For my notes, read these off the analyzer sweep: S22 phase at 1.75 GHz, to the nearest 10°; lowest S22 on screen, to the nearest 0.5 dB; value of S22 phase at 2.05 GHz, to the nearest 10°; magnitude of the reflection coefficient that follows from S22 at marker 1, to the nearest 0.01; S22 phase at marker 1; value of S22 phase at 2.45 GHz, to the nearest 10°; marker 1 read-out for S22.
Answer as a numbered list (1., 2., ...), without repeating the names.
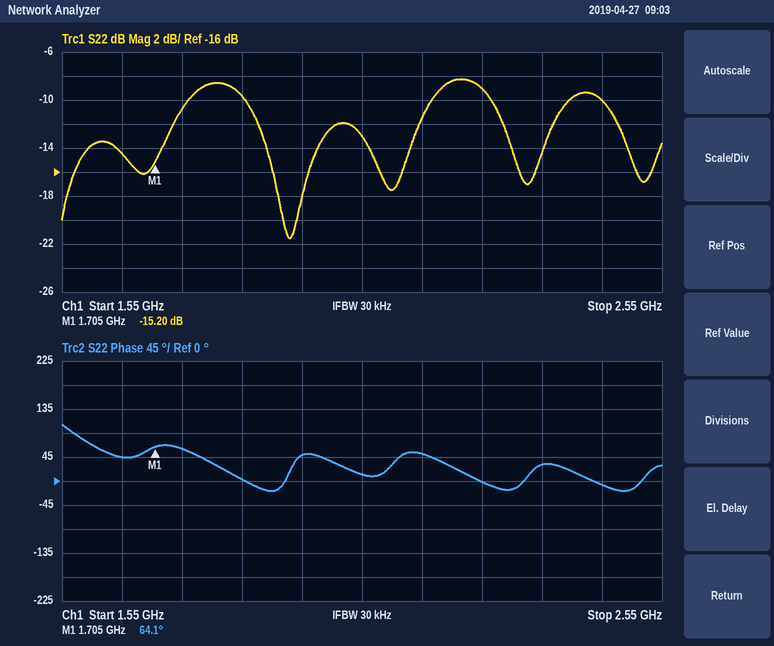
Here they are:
1. 60°
2. -21.5 dB
3. 10°
4. 0.17
5. 64.1°
6. -10°
7. -15.20 dB
